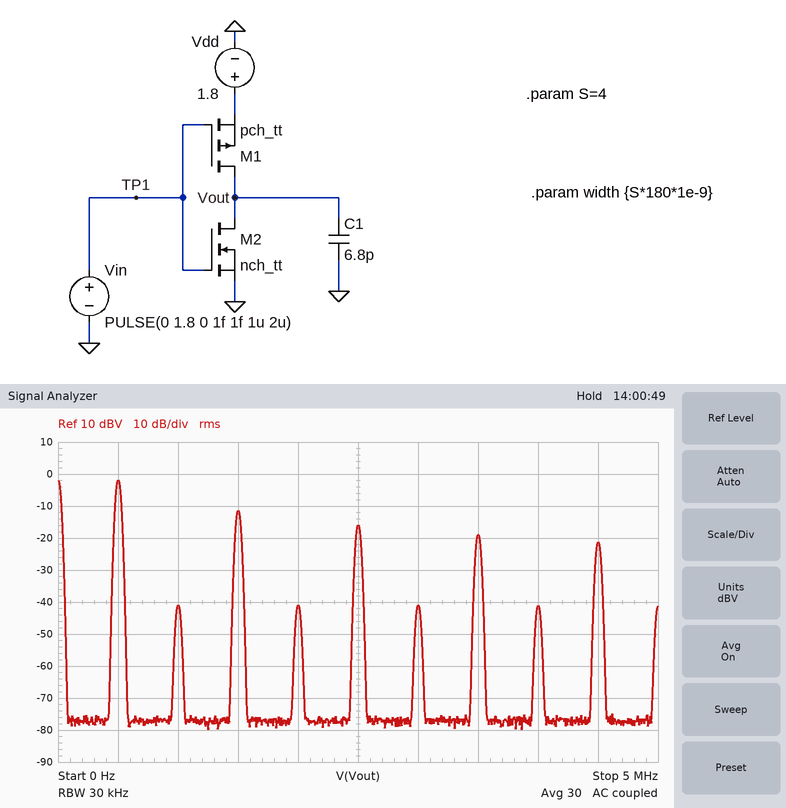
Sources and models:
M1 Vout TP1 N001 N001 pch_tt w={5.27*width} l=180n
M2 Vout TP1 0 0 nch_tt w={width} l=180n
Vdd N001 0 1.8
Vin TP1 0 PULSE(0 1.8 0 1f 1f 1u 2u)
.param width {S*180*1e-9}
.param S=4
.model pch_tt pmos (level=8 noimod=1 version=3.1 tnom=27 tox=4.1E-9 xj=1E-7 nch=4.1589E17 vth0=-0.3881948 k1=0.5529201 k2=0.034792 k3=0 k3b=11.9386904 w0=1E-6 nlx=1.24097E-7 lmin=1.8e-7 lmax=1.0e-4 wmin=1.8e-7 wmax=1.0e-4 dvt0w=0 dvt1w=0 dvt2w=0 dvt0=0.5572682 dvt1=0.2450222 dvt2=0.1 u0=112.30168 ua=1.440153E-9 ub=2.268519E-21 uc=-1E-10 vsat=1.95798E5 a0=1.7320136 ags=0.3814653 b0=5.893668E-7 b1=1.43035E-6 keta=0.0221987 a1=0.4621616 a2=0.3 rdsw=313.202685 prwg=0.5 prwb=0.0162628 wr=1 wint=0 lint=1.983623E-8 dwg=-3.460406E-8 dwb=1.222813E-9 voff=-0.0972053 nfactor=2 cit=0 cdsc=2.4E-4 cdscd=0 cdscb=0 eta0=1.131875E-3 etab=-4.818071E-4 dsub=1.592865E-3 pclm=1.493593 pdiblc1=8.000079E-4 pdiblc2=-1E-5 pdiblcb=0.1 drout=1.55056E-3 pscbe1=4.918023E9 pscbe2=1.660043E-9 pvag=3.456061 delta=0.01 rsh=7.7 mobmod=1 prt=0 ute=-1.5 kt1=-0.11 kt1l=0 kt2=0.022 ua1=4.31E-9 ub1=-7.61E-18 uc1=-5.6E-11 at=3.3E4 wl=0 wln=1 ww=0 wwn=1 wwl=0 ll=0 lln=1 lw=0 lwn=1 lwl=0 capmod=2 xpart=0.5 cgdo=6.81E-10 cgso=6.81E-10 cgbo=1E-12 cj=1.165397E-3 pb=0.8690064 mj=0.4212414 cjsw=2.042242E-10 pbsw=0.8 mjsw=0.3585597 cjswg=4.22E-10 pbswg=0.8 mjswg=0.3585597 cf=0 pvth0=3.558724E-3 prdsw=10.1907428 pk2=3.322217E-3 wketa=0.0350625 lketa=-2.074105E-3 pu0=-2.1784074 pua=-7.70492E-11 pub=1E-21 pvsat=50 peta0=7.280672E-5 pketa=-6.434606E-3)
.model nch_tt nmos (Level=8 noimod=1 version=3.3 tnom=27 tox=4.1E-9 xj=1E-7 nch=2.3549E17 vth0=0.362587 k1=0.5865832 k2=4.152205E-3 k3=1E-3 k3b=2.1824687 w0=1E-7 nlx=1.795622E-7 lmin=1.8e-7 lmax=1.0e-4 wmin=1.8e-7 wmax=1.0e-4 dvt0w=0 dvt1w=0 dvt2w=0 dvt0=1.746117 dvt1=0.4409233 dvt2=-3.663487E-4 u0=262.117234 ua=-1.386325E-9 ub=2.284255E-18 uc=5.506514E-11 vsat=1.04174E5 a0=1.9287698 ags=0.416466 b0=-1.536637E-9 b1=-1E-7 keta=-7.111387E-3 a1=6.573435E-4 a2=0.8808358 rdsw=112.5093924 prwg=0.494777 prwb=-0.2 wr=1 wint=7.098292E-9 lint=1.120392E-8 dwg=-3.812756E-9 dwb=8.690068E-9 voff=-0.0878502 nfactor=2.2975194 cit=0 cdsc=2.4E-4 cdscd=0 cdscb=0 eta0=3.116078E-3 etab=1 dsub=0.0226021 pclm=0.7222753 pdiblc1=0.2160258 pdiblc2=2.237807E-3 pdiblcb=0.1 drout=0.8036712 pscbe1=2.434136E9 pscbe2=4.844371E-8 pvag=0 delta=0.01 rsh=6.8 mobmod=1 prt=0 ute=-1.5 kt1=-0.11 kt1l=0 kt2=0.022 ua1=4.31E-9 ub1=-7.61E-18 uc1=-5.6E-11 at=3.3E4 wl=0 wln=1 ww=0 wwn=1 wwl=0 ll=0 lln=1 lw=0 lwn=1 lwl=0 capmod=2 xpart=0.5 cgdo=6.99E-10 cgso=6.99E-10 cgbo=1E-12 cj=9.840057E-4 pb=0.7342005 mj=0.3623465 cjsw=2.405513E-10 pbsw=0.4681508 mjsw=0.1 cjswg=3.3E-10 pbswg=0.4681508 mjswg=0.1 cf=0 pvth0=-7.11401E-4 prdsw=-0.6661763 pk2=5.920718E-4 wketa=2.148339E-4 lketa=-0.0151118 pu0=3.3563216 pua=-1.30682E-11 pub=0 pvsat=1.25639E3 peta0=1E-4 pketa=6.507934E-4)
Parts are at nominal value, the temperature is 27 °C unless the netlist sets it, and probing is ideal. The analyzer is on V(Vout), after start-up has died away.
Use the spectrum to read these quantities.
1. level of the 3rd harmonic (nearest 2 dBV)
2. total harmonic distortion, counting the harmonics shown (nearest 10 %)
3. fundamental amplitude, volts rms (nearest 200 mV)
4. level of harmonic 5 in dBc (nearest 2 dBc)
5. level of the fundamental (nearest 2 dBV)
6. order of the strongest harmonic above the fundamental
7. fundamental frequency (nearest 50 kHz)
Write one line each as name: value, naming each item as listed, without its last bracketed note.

level of the 3rd harmonic: -12 dBV
total harmonic distortion, counting the harmonics shown: 40 %
fundamental amplitude, volts rms: 800 mV
level of harmonic 5 in dBc: -14 dBc
level of the fundamental: -2 dBV
order of the strongest harmonic above the fundamental: 3
fundamental frequency: 500 kHz
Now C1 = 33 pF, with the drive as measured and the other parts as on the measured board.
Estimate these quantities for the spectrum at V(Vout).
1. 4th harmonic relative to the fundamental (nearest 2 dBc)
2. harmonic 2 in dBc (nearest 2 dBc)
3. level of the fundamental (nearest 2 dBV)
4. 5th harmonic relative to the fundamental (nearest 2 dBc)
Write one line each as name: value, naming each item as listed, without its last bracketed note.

4th harmonic relative to the fundamental: -26 dBc
harmonic 2 in dBc: -26 dBc
level of the fundamental: -2 dBV
5th harmonic relative to the fundamental: -16 dBc
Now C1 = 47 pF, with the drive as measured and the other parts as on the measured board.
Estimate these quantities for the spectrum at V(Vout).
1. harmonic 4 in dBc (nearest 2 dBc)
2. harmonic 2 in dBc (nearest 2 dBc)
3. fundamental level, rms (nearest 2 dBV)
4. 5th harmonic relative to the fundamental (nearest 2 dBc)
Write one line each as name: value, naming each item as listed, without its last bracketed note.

harmonic 4 in dBc: -24 dBc
harmonic 2 in dBc: -22 dBc
fundamental level, rms: -2 dBV
5th harmonic relative to the fundamental: -18 dBc
